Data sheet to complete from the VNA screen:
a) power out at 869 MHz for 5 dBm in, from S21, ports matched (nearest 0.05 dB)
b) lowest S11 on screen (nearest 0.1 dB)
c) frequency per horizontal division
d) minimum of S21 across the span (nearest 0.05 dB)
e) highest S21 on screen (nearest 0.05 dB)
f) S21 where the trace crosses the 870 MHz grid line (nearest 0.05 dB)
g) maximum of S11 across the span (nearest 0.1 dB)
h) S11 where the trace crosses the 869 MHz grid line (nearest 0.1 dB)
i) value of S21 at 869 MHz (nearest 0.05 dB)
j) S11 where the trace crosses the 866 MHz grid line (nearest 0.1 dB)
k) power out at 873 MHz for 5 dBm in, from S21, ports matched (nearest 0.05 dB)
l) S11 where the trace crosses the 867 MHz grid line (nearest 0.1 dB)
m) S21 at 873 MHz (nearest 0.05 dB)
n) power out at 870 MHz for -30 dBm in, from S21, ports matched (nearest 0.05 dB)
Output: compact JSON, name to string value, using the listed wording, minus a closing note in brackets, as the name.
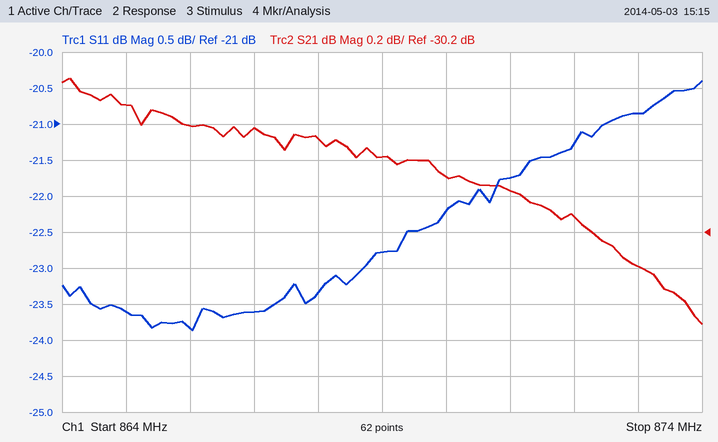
{"power out at 869 MHz for 5 dBm in, from S21, ports matched": "-24.80 dBm", "lowest S11 on screen": "-23.9 dB", "frequency per horizontal division": "1 MHz", "minimum of S21 across the span": "-30.70 dB", "highest S21 on screen": "-29.35 dB", "S21 where the trace crosses the 870 MHz grid line": "-29.90 dB", "maximum of S11 across the span": "-20.4 dB", "S11 where the trace crosses the 869 MHz grid line": "-22.8 dB", "value of S21 at 869 MHz": "-29.80 dB", "S11 where the trace crosses the 866 MHz grid line": "-23.8 dB", "power out at 873 MHz for 5 dBm in, from S21, ports matched": "-25.40 dBm", "S11 where the trace crosses the 867 MHz grid line": "-23.6 dB", "S21 at 873 MHz": "-30.40 dB", "power out at 870 MHz for -30 dBm in, from S21, ports matched": "-59.90 dBm"}
